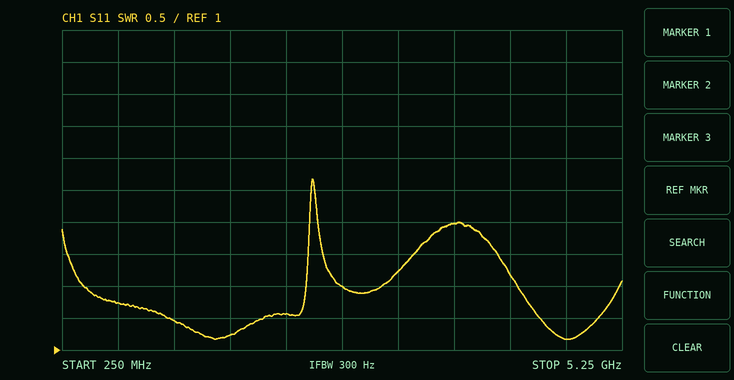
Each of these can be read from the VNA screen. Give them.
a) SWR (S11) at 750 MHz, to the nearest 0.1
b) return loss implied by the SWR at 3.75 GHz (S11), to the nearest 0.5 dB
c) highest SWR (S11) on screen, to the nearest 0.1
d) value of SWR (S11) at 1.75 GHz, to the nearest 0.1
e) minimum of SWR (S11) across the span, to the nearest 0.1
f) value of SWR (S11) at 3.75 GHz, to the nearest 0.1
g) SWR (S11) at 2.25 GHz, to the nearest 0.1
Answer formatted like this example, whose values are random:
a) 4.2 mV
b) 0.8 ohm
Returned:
a) 1.7
b) 6.0 dB
c) 3.7
d) 1.2
e) 1.2
f) 3.0
g) 1.6
